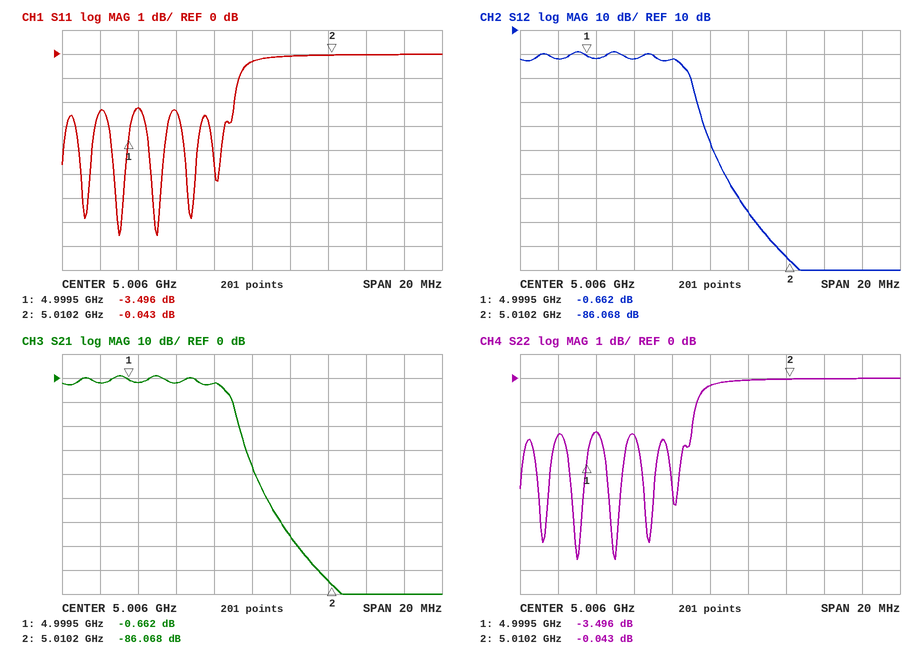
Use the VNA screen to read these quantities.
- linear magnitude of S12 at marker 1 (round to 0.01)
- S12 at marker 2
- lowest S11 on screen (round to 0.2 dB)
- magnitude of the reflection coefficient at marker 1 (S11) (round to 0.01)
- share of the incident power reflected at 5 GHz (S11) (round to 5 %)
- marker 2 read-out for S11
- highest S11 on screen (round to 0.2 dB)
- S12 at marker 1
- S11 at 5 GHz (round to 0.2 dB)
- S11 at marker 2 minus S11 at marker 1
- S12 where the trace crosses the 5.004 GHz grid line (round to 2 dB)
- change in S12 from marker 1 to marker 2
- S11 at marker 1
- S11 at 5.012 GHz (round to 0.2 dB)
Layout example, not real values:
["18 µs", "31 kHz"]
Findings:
["0.93", "-86.068 dB", "-7.6 dB", "0.67", "60 %", "-0.043 dB", "0.0 dB", "-0.662 dB", "-2.2 dB", "3.453 dB", "-2 dB", "-85.406 dB", "-3.496 dB", "0.0 dB"]
